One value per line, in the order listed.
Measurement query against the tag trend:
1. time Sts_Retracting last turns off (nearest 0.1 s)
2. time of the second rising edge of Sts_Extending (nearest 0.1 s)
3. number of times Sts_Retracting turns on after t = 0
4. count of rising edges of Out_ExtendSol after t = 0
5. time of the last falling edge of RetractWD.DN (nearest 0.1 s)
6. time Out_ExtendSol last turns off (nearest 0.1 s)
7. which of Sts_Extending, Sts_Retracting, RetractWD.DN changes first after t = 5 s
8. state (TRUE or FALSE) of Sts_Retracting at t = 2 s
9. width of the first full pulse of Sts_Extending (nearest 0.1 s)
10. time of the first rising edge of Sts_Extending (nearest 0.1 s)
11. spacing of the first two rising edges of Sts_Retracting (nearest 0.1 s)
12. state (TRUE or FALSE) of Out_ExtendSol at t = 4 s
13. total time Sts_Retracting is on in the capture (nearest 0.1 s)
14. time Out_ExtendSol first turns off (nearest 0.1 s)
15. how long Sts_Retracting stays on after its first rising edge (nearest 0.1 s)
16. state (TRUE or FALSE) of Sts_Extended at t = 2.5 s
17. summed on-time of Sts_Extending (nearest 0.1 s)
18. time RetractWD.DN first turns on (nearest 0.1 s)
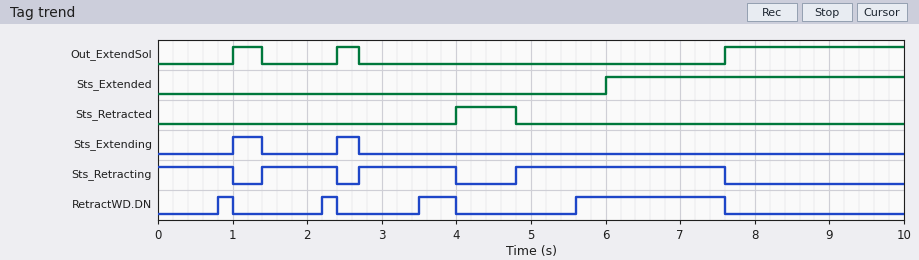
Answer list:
7.6 s
2.4 s
3
3
7.6 s
2.7 s
RetractWD.DN
TRUE
0.4 s
1.0 s
1.3 s
FALSE
6.1 s
1.4 s
1.0 s
FALSE
0.7 s
0.8 s
